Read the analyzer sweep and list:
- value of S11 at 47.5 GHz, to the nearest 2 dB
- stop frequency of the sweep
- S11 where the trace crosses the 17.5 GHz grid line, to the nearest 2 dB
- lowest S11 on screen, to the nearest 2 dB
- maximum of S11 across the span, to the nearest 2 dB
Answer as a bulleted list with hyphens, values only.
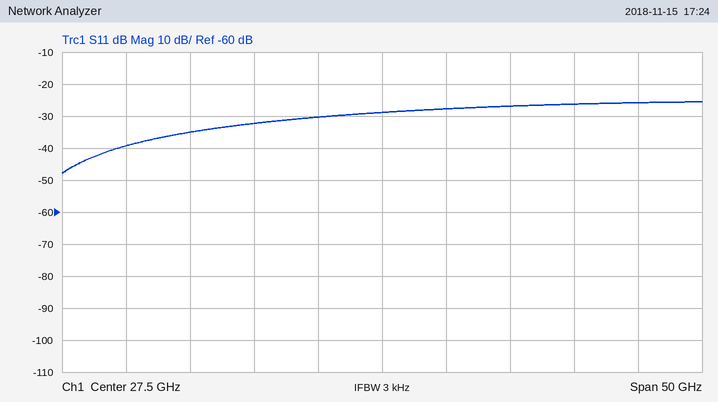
- -26 dB
- 52.5 GHz
- -32 dB
- -48 dB
- -26 dB
